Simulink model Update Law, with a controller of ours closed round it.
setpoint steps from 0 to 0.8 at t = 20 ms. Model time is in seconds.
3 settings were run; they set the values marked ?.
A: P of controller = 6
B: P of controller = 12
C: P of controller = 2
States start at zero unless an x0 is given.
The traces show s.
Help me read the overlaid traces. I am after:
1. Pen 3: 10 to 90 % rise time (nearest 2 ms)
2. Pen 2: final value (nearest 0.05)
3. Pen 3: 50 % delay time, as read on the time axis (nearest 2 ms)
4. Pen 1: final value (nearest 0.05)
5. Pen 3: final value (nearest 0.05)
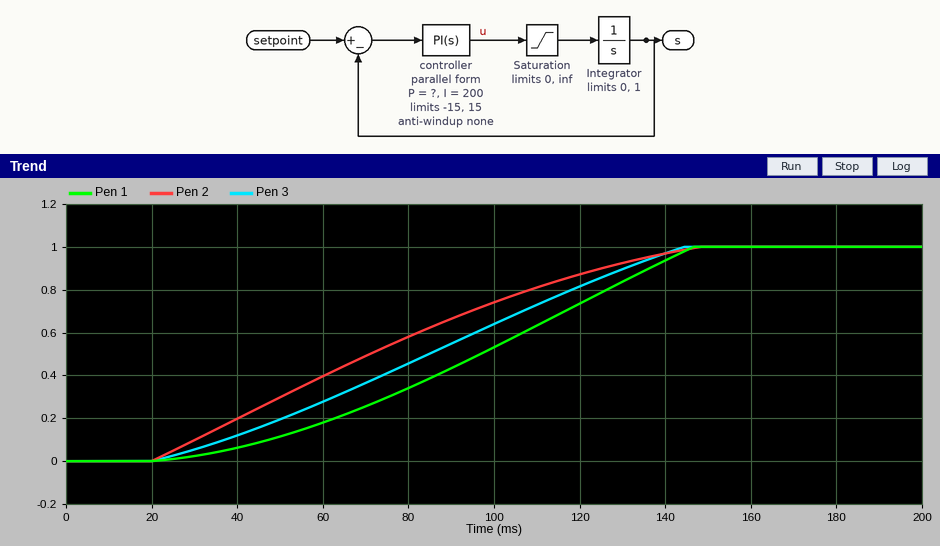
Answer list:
94 ms
1.00
84 ms
1.00
1.00
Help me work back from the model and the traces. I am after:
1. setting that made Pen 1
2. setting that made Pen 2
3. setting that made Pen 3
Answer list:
C
B
A
